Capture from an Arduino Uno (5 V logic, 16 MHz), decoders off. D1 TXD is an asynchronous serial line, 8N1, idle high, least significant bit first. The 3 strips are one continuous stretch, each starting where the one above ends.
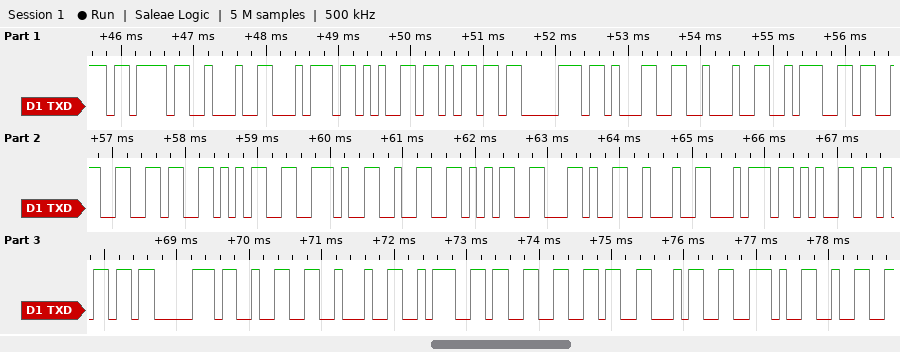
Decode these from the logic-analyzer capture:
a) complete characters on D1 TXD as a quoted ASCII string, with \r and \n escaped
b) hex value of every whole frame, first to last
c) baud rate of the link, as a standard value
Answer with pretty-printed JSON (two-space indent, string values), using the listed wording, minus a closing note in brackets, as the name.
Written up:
{
  "complete characters on D1 TXD as a quoted ASCII string, with \\r and \\n escaped": "\"{\\\"temp1\\\":365.25,\\\"temp2\\\":364.2\"",
  "hex value of every whole frame, first to last": "0x7B 0x22 0x74 0x65 0x6D 0x70 0x31 0x22 0x3A 0x33 0x36 0x35 0x2E 0x32 0x35 0x2C 0x22 0x74 0x65 0x6D 0x70 0x32 0x22 0x3A 0x33 0x36 0x34 0x2E 0x32",
  "baud rate of the link, as a standard value": "9600 baud"
}
